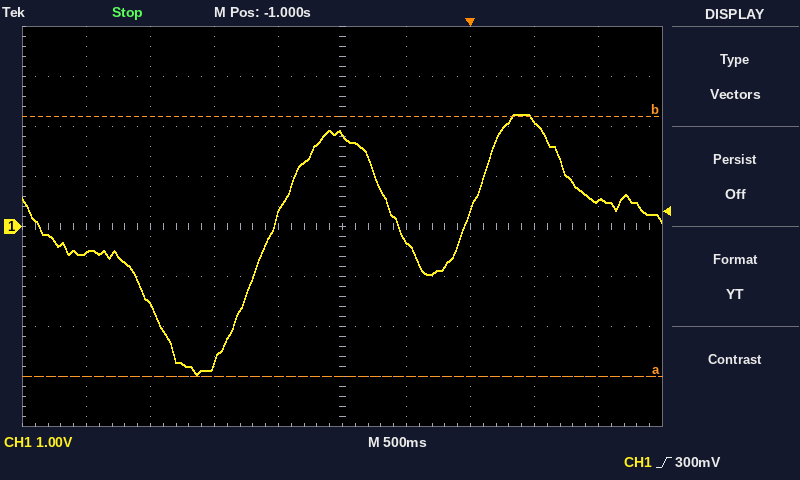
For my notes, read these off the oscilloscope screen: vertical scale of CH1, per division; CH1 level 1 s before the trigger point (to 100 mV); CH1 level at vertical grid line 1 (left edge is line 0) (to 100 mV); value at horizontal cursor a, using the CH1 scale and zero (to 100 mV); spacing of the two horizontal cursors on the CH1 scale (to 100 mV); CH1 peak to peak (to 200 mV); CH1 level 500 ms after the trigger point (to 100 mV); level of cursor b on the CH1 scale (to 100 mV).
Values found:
1 V
1.8 V
-500 mV
-3.0 V
5.2 V
5.2 V
2.1 V
2.2 V
